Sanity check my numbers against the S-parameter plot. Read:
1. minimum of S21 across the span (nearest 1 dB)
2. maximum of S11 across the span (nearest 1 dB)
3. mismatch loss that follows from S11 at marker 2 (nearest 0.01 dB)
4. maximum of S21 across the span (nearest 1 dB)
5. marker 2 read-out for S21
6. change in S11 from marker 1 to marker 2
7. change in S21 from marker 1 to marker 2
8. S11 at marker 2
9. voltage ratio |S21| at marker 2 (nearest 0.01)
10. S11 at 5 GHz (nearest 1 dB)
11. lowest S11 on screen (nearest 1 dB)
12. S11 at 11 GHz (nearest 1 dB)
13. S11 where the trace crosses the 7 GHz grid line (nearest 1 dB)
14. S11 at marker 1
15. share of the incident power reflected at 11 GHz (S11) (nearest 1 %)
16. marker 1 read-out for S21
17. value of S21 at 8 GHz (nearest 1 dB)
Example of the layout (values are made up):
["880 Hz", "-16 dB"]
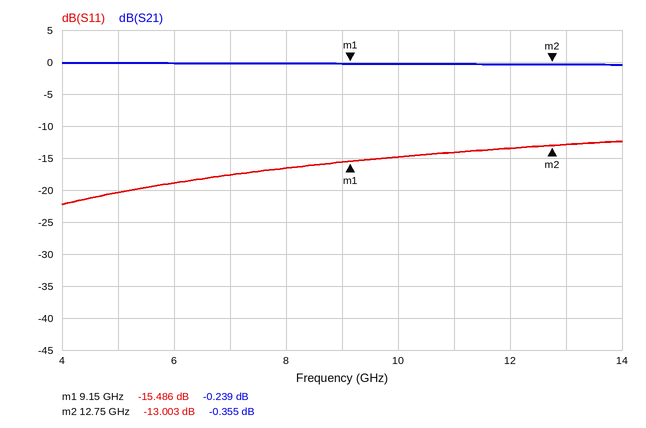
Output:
["0 dB", "-12 dB", "0.22 dB", "0 dB", "-0.355 dB", "2.483 dB", "-0.116 dB", "-13.003 dB", "0.96", "-20 dB", "-22 dB", "-14 dB", "-18 dB", "-15.486 dB", "4 %", "-0.239 dB", "0 dB"]
